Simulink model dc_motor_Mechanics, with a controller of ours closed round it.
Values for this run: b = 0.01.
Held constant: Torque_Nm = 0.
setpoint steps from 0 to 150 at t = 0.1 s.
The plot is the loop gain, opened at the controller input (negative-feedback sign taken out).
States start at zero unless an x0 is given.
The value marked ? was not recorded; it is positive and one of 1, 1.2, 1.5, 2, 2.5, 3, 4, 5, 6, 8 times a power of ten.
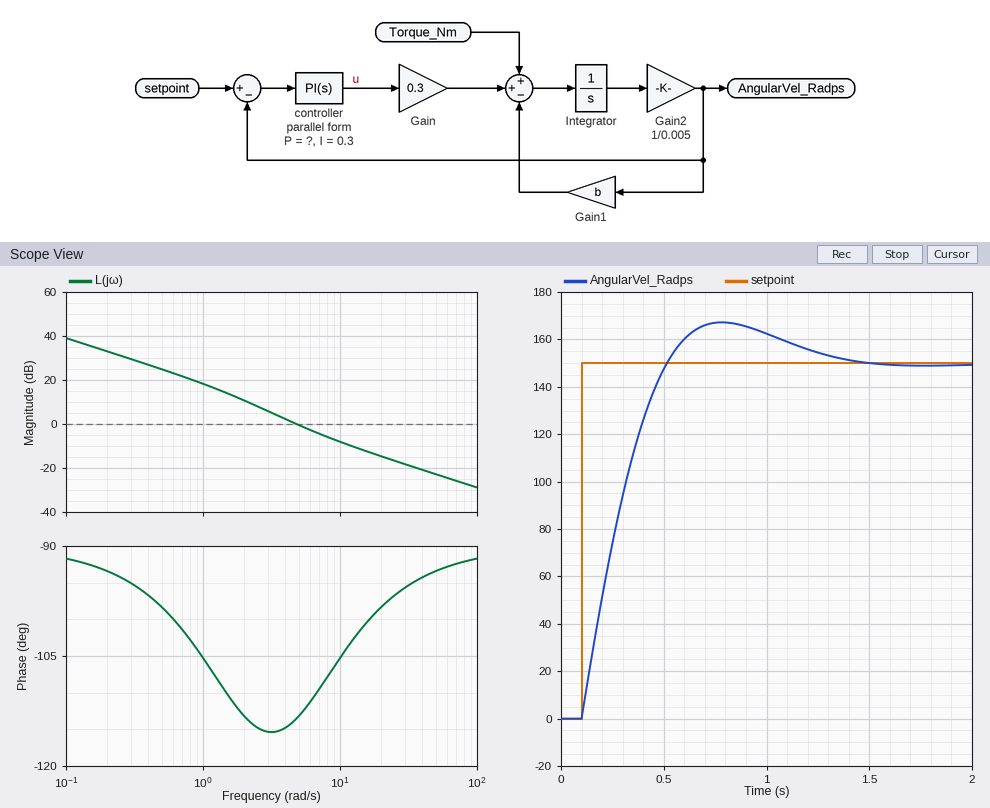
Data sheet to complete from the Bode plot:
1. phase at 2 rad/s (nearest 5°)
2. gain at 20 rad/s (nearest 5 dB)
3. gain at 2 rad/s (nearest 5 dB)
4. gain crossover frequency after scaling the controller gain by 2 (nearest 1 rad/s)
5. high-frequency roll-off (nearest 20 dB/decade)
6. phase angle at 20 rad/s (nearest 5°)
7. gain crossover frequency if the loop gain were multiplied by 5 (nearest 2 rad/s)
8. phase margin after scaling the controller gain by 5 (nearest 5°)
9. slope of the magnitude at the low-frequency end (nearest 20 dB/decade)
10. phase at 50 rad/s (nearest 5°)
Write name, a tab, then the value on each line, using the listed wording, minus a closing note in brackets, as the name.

phase at 2 rad/s	-115°
gain at 20 rad/s	-15 dB
gain at 2 rad/s	10 dB
gain crossover frequency after scaling the controller gain by 2	8 rad/s
high-frequency roll-off	-20 dB/decade
phase angle at 20 rad/s	-100°
gain crossover frequency if the loop gain were multiplied by 5	18 rad/s
phase margin after scaling the controller gain by 5	80°
slope of the magnitude at the low-frequency end	-20 dB/decade
phase at 50 rad/s	-95°
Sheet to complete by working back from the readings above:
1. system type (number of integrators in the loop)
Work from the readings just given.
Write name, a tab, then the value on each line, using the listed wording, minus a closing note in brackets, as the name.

system type	1
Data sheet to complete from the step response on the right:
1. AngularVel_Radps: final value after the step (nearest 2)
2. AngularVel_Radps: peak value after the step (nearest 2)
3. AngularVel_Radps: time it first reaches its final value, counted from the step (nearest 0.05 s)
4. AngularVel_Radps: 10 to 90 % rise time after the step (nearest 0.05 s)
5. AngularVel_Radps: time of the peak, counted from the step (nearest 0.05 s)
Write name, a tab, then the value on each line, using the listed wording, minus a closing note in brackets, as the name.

AngularVel_Radps: final value after the step	150
AngularVel_Radps: peak value after the step	168
AngularVel_Radps: time it first reaches its final value, counted from the step	0.40 s
AngularVel_Radps: 10 to 90 % rise time after the step	0.30 s
AngularVel_Radps: time of the peak, counted from the step	0.70 s
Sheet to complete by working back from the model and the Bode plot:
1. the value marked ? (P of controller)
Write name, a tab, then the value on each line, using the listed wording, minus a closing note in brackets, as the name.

the value marked ?	0.06
